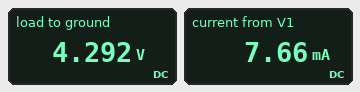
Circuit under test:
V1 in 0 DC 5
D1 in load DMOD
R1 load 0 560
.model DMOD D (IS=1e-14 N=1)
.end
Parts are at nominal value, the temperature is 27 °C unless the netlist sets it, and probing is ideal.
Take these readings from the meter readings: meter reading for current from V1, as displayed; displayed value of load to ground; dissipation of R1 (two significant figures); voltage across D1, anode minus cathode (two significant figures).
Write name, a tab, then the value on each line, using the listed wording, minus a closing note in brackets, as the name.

meter reading for current from V1, as displayed	7.66 mA
displayed value of load to ground	4.292 V
dissipation of R1	33 mW
voltage across D1, anode minus cathode	710 mV
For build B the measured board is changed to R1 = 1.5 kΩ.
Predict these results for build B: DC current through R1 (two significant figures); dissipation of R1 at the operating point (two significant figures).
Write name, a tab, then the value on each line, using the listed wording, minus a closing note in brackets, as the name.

DC current through R1	2.9 mA
dissipation of R1 at the operating point	12 mW
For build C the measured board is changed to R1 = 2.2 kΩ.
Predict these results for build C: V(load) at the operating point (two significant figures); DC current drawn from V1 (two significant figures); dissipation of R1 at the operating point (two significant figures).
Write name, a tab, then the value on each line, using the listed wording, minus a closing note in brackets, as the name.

V(load) at the operating point	4.3 V
DC current drawn from V1	2.0 mA
dissipation of R1 at the operating point	8.5 mW
